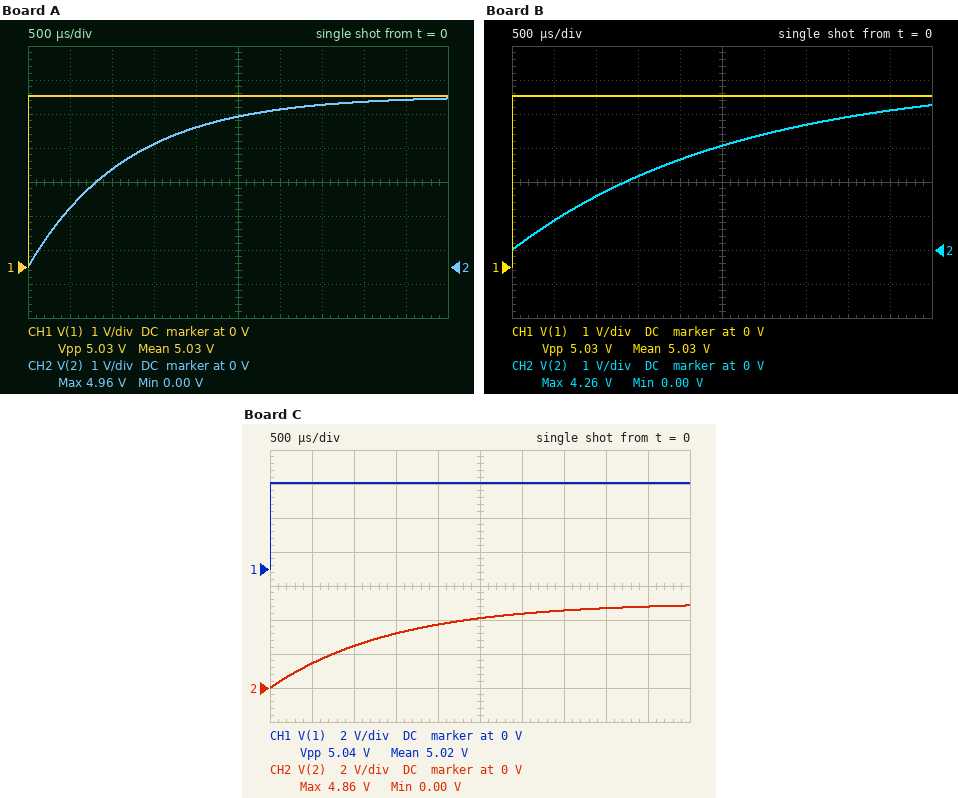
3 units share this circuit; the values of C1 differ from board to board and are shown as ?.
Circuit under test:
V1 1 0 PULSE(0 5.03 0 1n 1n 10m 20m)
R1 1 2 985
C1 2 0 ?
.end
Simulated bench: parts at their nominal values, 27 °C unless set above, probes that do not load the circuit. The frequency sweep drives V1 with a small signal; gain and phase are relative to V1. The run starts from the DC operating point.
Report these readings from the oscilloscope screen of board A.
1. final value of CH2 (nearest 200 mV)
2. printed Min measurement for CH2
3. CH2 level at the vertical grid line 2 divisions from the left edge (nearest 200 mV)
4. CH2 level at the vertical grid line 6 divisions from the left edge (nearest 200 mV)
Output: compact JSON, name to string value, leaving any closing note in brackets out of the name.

{"final value of CH2": "5.0 V", "printed Min measurement for CH2": "0.00 V", "CH2 level at the vertical grid line 2 divisions from the left edge": "2.8 V", "CH2 level at the vertical grid line 6 divisions from the left edge": "4.6 V"}
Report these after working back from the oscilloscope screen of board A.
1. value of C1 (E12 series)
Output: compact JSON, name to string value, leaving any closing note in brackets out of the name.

{"value of C1": "1.2 µF"}
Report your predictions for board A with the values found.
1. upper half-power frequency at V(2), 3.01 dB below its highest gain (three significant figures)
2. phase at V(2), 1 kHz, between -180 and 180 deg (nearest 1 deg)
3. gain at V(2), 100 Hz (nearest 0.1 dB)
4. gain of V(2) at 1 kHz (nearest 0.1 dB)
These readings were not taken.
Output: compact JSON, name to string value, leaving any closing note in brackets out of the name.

{"upper half-power frequency at V(2), 3.01 dB below its highest gain": "135 Hz", "phase at V(2), 1 kHz, between -180 and 180 deg": "-82 deg", "gain at V(2), 100 Hz": "-1.9 dB", "gain of V(2) at 1 kHz": "-17.5 dB"}
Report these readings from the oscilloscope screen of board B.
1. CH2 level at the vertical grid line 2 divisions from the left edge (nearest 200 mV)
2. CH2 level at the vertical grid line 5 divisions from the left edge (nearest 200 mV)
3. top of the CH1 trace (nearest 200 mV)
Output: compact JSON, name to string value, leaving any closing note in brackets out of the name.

{"CH2 level at the vertical grid line 2 divisions from the left edge": "1.6 V", "CH2 level at the vertical grid line 5 divisions from the left edge": "3.0 V", "top of the CH1 trace": "5.0 V"}
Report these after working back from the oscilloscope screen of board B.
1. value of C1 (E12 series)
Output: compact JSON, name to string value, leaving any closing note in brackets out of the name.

{"value of C1": "2.7 µF"}
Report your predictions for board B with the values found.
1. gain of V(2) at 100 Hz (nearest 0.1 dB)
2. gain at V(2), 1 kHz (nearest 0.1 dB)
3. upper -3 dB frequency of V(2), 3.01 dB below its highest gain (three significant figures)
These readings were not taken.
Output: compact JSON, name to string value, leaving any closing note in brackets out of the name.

{"gain of V(2) at 100 Hz": "-5.8 dB", "gain at V(2), 1 kHz": "-24.5 dB", "upper -3 dB frequency of V(2), 3.01 dB below its highest gain": "59.8 Hz"}
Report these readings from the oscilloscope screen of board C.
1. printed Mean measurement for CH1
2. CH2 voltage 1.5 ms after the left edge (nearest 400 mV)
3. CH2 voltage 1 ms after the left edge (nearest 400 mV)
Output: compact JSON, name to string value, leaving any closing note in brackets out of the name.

{"printed Mean measurement for CH1": "5.02 V", "CH2 voltage 1.5 ms after the left edge": "3.2 V", "CH2 voltage 1 ms after the left edge": "2.4 V"}
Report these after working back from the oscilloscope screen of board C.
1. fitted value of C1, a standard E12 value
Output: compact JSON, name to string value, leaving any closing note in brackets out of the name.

{"fitted value of C1, a standard E12 value": "1.5 µF"}
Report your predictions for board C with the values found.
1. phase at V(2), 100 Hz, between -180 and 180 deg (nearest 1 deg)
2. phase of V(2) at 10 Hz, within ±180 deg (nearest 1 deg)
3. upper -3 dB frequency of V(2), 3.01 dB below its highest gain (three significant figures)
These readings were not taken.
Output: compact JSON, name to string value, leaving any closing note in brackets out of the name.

{"phase at V(2), 100 Hz, between -180 and 180 deg": "-43 deg", "phase of V(2) at 10 Hz, within ±180 deg": "-5 deg", "upper -3 dB frequency of V(2), 3.01 dB below its highest gain": "108 Hz"}
